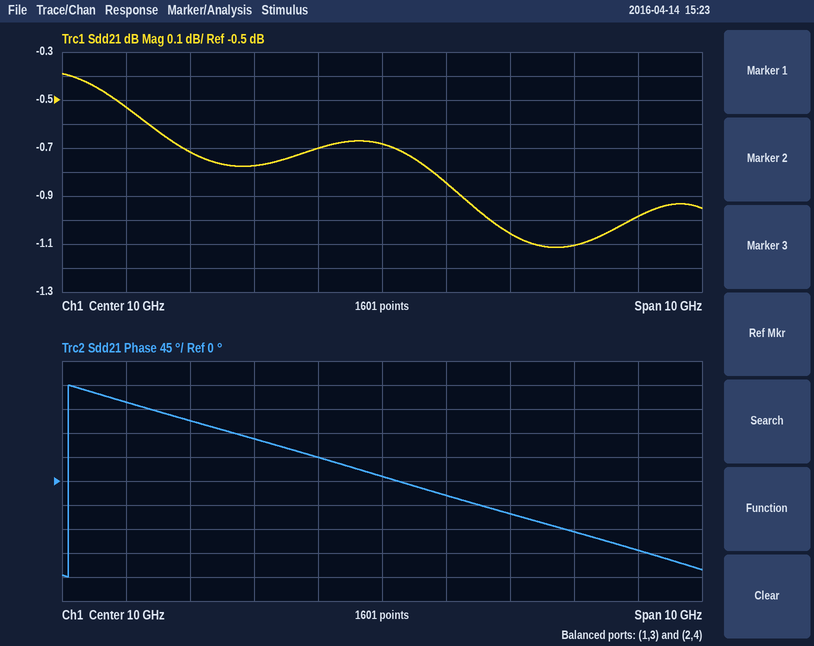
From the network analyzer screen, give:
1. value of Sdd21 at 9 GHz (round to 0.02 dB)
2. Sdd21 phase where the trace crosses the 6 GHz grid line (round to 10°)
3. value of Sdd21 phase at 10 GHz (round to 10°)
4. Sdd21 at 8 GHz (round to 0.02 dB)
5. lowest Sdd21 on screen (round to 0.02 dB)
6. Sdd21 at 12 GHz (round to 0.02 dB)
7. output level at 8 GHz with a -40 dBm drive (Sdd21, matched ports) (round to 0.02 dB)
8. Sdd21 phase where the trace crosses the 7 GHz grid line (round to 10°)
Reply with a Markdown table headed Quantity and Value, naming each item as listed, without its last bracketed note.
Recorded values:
| Quantity | Value |
|---|---|
| value of Sdd21 at 9 GHz | -0.70 dB |
| Sdd21 phase where the trace crosses the 6 GHz grid line | 150° |
| value of Sdd21 phase at 10 GHz | 10° |
| Sdd21 at 8 GHz | -0.78 dB |
| lowest Sdd21 on screen | -1.12 dB |
| Sdd21 at 12 GHz | -1.06 dB |
| output level at 8 GHz with a -40 dBm drive (Sdd21, matched ports) | -40.78 dBm |
| Sdd21 phase where the trace crosses the 7 GHz grid line | 110° |
